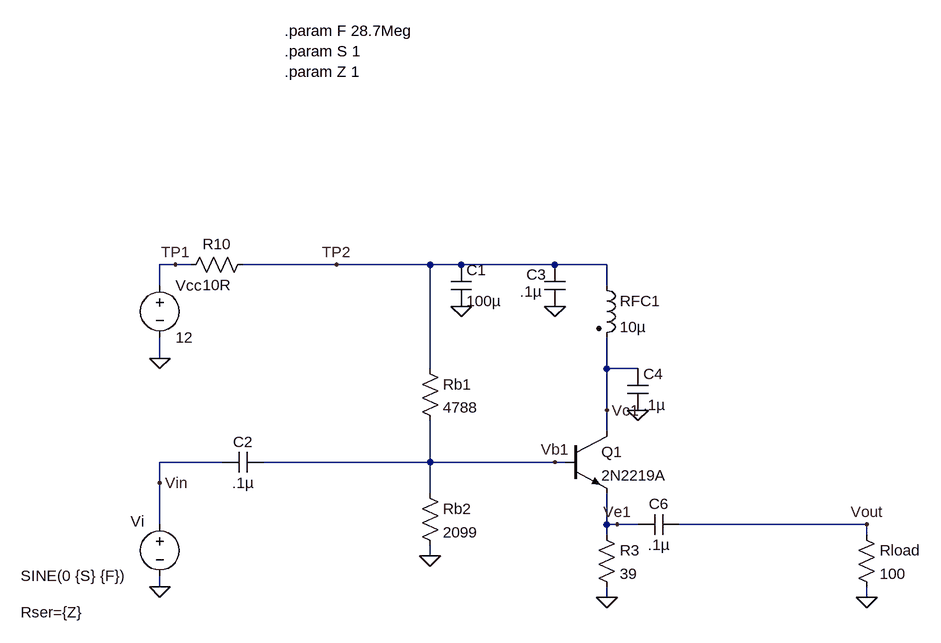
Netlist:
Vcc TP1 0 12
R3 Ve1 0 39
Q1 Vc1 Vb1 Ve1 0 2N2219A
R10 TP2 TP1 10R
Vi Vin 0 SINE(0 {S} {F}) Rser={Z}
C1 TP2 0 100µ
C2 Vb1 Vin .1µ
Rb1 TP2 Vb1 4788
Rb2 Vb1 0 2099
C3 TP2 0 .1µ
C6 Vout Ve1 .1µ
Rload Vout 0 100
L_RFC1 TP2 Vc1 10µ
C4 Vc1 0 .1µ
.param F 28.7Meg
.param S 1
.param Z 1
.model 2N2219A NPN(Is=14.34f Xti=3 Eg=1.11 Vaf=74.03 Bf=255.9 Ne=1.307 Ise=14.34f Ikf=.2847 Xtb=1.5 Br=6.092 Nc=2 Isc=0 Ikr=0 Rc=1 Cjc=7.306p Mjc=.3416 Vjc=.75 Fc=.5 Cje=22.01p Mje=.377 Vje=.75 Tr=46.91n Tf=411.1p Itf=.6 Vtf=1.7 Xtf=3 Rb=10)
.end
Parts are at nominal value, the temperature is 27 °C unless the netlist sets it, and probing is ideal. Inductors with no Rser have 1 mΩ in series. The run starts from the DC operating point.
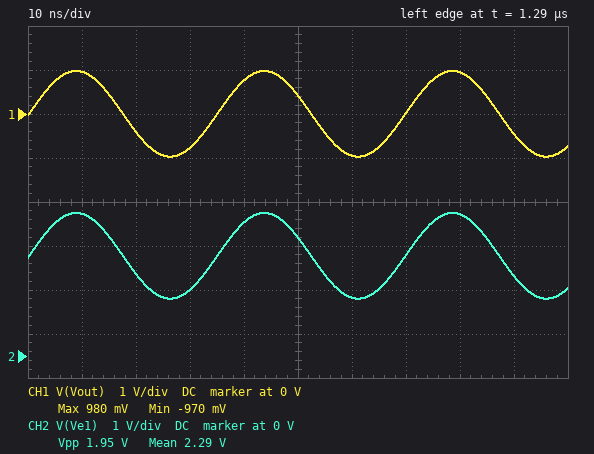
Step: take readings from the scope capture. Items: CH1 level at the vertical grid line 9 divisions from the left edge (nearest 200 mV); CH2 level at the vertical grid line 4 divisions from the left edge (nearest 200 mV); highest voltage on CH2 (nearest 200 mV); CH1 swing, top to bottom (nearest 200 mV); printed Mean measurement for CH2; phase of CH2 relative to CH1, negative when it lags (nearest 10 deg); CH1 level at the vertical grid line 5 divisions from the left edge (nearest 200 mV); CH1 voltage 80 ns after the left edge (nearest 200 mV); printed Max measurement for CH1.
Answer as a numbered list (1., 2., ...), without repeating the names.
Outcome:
1. -400 mV
2. 3.0 V
3. 3.2 V
4. 2.0 V
5. 2.29 V
6. 0 deg
7. 400 mV
8. 1.0 V
9. 980 mV
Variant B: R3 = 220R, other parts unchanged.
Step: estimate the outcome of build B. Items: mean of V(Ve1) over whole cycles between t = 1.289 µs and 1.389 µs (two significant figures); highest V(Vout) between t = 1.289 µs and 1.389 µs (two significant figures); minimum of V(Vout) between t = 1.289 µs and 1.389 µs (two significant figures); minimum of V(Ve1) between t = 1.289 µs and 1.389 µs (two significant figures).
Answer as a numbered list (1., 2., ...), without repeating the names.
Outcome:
1. 2.8 V
2. 970 mV
3. -900 mV
4. 1.9 V
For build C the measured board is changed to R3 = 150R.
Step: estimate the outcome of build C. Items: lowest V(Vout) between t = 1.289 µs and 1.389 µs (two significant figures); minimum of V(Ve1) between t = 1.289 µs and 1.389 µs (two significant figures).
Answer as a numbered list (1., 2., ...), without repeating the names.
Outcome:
1. -950 mV
2. 1.8 V
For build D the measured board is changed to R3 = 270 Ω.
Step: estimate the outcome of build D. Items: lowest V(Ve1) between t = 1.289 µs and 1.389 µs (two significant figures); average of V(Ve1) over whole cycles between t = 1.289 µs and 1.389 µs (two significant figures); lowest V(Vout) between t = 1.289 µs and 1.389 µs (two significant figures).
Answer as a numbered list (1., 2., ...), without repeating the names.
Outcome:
1. 2.0 V
2. 2.9 V
3. -850 mV
